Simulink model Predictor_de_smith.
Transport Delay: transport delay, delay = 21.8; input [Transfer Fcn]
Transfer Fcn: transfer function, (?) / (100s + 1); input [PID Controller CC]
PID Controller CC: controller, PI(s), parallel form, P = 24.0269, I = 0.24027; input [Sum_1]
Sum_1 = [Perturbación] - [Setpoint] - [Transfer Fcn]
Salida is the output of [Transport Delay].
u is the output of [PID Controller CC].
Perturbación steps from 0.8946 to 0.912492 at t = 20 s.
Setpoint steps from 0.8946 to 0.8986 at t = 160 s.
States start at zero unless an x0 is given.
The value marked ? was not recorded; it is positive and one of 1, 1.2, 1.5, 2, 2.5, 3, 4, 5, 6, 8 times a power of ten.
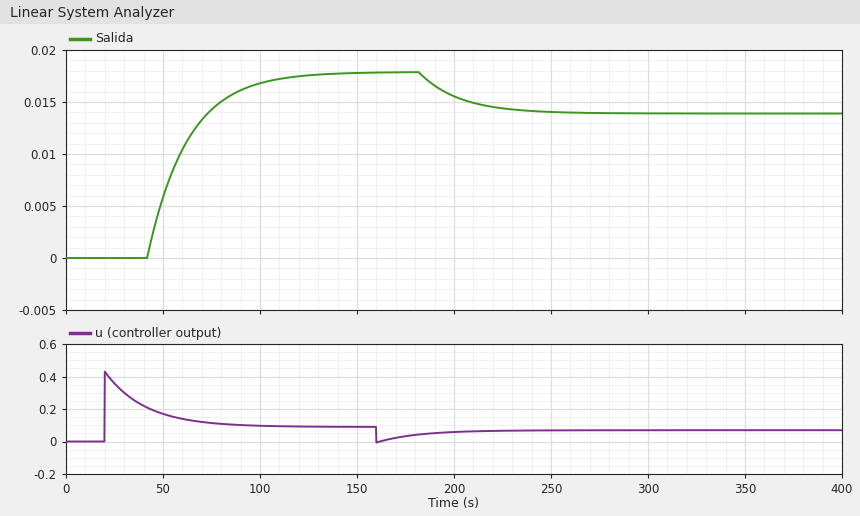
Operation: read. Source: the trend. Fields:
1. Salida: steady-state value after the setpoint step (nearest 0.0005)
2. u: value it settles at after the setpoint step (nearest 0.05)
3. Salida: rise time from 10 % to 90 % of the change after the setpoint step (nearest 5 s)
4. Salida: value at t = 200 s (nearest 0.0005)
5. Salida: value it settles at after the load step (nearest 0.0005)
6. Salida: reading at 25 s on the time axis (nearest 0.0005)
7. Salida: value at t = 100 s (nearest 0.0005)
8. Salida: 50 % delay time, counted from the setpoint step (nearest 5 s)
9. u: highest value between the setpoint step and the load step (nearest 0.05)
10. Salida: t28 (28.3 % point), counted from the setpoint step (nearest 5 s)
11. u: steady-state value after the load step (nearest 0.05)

0.0180
0.10
45 s
0.0155
0.0140
0.0000
0.0170
35 s
0.45
30 s
0.05
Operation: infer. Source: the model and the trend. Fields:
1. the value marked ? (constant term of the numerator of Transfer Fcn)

0.2
